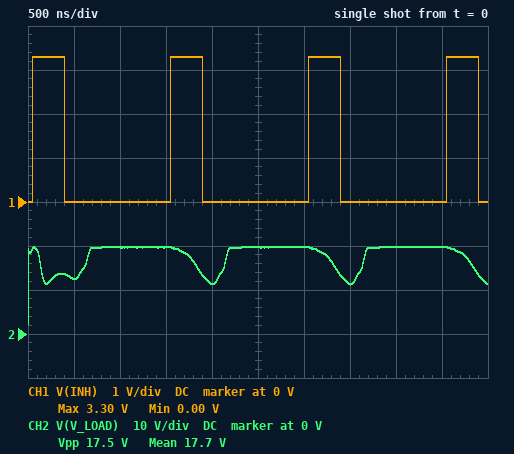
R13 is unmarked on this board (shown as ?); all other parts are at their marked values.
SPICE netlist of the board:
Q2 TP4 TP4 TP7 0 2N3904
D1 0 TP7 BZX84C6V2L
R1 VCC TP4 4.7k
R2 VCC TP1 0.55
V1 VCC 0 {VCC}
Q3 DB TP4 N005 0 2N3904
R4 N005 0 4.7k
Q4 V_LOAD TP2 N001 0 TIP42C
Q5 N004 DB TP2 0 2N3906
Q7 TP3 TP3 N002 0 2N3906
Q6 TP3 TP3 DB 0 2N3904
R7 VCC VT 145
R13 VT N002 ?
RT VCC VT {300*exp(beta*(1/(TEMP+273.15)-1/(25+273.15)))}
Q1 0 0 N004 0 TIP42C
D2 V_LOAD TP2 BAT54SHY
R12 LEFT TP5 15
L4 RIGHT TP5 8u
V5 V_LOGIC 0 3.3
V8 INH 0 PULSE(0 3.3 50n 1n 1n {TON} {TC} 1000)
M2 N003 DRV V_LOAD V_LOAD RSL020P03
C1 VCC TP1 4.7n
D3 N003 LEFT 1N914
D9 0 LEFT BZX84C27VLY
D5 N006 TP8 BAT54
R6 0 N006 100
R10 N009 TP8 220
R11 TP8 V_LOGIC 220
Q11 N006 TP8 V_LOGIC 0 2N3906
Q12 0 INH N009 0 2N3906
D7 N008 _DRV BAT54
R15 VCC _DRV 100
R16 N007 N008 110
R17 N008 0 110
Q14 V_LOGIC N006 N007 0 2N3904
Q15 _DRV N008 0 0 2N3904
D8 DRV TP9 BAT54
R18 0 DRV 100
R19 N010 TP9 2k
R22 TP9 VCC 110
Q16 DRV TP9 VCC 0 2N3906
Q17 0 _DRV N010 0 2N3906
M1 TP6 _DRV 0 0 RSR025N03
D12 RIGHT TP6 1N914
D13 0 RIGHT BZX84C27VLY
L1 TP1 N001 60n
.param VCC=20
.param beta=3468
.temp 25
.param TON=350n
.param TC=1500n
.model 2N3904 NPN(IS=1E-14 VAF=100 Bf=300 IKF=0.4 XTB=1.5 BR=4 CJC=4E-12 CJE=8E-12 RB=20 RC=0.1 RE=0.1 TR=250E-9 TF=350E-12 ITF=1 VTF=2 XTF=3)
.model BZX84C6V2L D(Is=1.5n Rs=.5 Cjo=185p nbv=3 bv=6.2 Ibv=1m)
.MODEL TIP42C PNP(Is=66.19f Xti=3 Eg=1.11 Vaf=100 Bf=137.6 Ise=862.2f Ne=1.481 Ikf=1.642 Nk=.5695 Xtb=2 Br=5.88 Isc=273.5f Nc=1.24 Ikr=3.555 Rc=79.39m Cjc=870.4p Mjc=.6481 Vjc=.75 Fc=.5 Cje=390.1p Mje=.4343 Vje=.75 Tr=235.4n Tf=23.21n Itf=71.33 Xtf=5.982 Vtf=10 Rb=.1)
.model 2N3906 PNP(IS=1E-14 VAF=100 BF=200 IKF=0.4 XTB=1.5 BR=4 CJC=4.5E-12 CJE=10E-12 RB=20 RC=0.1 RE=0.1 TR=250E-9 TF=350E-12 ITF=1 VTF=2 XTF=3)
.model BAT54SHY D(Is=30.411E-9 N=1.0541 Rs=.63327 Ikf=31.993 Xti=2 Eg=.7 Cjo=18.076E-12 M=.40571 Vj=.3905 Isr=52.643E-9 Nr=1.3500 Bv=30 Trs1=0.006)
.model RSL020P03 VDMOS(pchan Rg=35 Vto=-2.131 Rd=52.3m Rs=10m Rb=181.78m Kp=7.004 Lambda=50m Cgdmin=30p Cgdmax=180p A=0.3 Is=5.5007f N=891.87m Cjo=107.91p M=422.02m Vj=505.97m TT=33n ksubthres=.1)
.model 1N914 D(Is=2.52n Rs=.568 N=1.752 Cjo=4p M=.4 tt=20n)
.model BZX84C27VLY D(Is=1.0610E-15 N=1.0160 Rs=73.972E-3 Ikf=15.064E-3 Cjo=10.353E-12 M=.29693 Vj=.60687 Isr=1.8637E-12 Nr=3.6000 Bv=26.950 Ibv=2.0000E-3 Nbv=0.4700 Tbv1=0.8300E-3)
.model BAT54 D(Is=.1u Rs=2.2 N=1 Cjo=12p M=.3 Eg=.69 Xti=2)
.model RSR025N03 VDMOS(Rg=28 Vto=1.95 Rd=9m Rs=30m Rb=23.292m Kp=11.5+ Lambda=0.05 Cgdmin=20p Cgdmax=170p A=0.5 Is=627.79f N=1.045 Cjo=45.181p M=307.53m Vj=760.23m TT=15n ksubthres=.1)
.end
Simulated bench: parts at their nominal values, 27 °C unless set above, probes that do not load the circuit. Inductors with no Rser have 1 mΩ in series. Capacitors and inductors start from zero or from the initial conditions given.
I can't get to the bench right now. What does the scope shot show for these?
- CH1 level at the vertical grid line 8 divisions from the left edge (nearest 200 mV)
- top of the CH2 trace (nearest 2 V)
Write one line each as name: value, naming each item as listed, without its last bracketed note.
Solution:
CH1 level at the vertical grid line 8 divisions from the left edge: 0 V
top of the CH2 trace: 20 V
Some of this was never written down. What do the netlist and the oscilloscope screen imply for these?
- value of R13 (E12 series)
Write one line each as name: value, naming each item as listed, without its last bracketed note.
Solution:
value of R13: 220 Ω
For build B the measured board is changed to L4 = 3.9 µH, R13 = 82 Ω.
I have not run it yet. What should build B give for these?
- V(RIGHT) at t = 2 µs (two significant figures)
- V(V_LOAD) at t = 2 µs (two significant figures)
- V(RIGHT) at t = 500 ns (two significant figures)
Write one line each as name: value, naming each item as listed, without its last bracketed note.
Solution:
V(RIGHT) at t = 2 µs: 980 mV
V(V_LOAD) at t = 2 µs: 5.8 V
V(RIGHT) at t = 500 ns: 960 mV
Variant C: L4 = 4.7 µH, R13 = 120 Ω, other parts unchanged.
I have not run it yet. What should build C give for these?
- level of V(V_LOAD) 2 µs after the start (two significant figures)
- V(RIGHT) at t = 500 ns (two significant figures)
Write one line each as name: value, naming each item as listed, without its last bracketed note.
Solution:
level of V(V_LOAD) 2 µs after the start: 6.9 V
V(RIGHT) at t = 500 ns: 1.0 V
